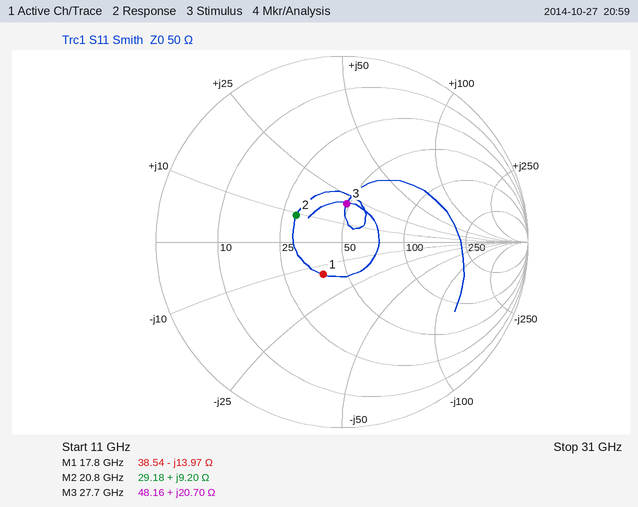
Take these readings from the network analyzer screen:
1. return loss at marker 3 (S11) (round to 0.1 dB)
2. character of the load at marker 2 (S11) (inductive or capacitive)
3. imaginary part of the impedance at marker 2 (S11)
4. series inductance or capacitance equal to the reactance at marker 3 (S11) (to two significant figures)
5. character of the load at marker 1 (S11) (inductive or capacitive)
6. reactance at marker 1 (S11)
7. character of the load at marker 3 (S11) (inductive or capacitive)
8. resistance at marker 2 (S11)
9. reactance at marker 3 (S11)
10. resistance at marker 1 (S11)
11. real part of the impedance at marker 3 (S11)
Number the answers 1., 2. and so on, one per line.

1. 13.7 dB
2. inductive
3. +9.20 Ω
4. 120 pH
5. capacitive
6. -13.97 Ω
7. inductive
8. 29.18 Ω
9. +20.70 Ω
10. 38.54 Ω
11. 48.16 Ω
